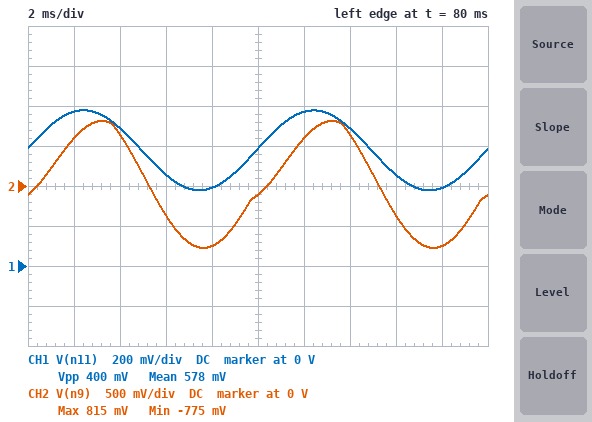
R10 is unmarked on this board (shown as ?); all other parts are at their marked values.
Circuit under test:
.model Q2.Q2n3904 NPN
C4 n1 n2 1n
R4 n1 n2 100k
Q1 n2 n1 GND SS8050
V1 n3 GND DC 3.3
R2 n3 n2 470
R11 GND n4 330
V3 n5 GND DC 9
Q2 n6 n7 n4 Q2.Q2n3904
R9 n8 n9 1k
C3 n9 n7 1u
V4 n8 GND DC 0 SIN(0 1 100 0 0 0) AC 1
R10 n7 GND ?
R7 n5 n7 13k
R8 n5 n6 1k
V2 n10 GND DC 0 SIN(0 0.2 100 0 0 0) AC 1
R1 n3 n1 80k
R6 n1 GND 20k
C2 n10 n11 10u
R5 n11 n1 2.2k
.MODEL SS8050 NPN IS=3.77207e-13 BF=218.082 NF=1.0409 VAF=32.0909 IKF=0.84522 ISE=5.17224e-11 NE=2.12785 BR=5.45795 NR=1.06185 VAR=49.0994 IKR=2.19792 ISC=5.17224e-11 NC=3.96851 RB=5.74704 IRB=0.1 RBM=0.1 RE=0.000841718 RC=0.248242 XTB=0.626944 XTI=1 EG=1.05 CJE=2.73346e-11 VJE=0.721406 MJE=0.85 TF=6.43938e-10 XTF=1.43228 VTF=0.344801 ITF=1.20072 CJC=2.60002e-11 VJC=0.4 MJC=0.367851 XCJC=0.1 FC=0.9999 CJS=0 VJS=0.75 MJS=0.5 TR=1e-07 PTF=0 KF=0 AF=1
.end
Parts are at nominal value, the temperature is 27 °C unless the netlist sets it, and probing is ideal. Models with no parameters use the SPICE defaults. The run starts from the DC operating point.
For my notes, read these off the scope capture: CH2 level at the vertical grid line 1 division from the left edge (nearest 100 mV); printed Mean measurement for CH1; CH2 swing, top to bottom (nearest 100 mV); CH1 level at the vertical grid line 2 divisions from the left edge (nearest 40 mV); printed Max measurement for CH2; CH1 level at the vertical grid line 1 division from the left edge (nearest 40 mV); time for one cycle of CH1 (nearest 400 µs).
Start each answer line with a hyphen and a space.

- 600 mV
- 578 mV
- 1.6 V
- 680 mV
- 815 mV
- 760 mV
- 10.0 ms
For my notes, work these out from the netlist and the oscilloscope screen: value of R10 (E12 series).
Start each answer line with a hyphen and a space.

- 8.2 kΩ
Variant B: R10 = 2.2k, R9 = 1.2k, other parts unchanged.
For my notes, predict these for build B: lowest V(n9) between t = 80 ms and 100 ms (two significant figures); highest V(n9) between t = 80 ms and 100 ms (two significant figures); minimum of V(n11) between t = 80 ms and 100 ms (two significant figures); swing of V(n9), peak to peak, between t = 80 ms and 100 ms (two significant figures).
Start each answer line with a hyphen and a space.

- -710 mV
- 710 mV
- 380 mV
- 1.4 V
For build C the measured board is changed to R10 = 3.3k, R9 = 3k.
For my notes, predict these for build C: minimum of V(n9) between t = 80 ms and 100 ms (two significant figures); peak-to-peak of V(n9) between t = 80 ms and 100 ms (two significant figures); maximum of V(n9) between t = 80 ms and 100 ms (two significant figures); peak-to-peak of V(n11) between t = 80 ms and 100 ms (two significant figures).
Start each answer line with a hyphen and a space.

- -510 mV
- 1.0 V
- 510 mV
- 400 mV
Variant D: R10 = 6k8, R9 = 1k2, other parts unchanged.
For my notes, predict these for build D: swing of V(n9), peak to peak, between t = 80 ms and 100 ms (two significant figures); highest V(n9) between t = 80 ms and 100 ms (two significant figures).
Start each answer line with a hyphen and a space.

- 1.5 V
- 780 mV
